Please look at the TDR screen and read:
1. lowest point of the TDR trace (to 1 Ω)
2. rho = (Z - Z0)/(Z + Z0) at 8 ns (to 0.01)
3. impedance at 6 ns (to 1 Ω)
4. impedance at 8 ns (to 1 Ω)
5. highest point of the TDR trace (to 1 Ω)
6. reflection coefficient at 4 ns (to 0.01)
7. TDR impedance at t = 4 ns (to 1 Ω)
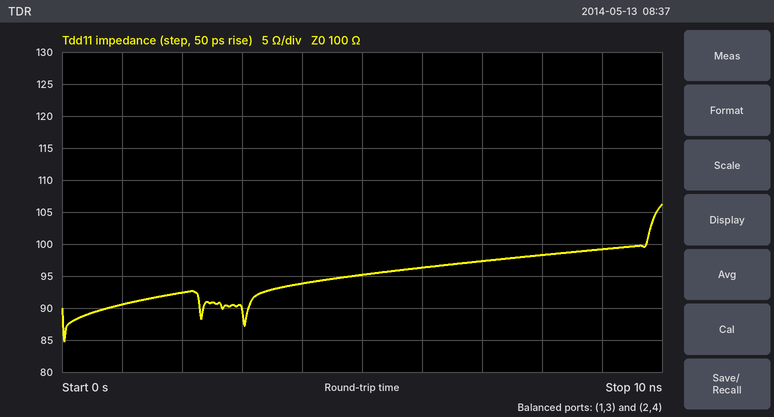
85 Ω
-0.01
96 Ω
98 Ω
106 Ω
-0.03
94 Ω
